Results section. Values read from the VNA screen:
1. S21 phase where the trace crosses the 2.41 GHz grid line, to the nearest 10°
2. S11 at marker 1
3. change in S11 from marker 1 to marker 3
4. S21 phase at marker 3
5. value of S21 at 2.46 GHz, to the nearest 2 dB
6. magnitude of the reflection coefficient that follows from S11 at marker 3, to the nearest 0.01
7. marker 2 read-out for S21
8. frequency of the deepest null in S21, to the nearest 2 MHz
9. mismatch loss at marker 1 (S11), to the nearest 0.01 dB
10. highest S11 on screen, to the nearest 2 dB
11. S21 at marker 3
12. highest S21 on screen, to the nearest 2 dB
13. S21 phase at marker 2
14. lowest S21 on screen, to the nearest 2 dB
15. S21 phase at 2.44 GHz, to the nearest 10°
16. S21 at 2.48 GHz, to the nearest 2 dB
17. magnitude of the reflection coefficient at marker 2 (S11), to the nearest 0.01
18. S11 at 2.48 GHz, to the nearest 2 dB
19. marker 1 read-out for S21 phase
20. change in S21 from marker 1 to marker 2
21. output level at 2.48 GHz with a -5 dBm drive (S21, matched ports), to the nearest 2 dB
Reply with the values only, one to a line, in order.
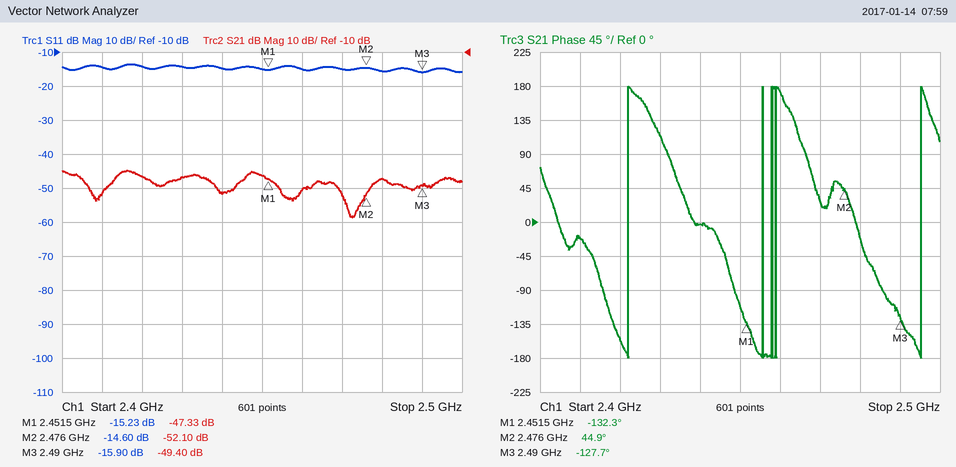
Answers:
-20°
-15.23 dB
-0.67 dB
-127.7°
-50 dB
0.16
-52.10 dB
2.472 GHz
0.13 dB
-14 dB
-49.40 dB
-44 dB
44.9°
-58 dB
0°
-48 dB
0.19
-16 dB
-132.3°
-4.77 dB
-52 dBm
